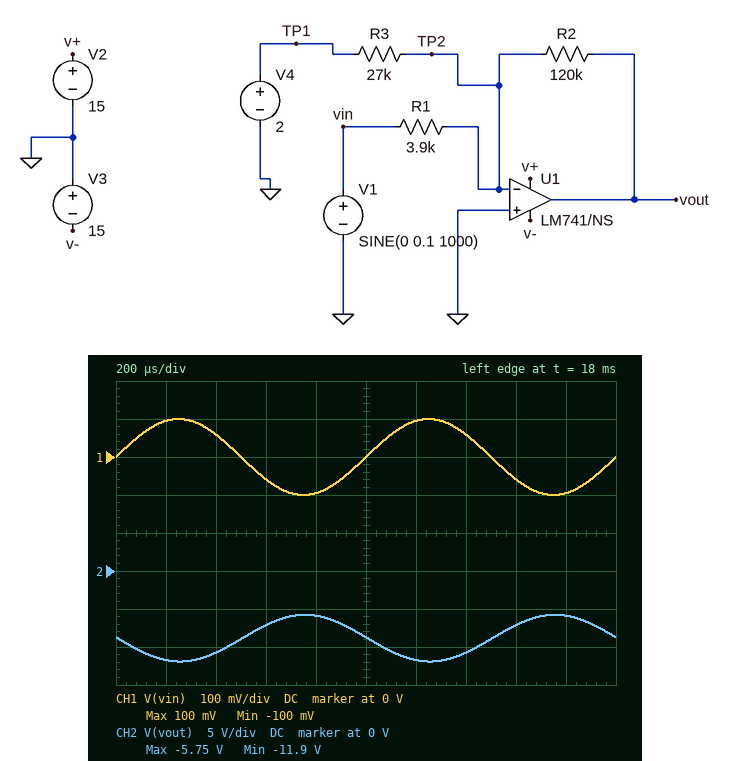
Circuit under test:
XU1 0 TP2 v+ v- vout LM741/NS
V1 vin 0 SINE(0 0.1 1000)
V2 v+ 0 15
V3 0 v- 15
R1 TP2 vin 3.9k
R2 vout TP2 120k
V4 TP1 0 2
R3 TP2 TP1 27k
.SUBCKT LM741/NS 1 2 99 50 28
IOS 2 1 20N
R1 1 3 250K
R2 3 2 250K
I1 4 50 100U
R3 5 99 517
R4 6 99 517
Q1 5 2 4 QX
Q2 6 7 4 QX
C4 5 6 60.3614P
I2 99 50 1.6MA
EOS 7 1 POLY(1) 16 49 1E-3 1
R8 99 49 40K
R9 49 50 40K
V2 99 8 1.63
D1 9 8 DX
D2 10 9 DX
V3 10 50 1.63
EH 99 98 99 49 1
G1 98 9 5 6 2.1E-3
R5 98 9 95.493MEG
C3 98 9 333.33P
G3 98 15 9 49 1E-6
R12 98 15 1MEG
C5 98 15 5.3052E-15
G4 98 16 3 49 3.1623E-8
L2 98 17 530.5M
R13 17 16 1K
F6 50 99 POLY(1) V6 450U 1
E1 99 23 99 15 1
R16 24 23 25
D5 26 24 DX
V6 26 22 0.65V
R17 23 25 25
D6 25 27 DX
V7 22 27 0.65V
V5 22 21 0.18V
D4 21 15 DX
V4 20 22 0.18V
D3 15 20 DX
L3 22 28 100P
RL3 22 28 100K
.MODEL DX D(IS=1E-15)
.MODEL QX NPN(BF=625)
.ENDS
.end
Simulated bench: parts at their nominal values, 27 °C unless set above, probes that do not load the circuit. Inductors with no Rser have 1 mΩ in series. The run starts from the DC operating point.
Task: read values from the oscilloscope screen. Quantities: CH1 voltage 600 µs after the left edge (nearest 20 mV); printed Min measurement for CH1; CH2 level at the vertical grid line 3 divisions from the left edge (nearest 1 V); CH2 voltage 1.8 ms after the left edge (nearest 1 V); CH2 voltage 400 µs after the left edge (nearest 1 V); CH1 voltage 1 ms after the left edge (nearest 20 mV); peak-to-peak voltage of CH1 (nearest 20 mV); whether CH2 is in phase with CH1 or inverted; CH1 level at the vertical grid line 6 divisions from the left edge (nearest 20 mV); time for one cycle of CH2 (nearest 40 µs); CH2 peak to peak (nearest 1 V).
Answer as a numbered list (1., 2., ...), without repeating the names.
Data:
1. -60 mV
2. -100 mV
3. -7 V
4. -6 V
5. -11 V
6. 0 V
7. 200 mV
8. inverted
9. 100 mV
10. 1.00 ms
11. 6 V
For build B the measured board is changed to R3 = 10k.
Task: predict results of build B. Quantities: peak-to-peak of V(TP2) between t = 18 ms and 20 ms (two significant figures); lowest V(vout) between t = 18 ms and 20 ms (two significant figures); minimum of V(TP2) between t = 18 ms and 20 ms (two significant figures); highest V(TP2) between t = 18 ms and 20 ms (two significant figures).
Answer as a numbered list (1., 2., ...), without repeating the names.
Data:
1. 140 mV
2. -14 V
3. 160 mV
4. 300 mV
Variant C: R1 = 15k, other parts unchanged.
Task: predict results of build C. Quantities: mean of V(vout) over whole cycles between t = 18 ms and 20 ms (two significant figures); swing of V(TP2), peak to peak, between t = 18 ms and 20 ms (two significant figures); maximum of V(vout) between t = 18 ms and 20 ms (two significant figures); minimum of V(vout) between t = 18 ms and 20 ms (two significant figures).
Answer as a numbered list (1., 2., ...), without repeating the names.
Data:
1. -8.9 V
2. 1.6 mV
3. -8.1 V
4. -9.7 V
